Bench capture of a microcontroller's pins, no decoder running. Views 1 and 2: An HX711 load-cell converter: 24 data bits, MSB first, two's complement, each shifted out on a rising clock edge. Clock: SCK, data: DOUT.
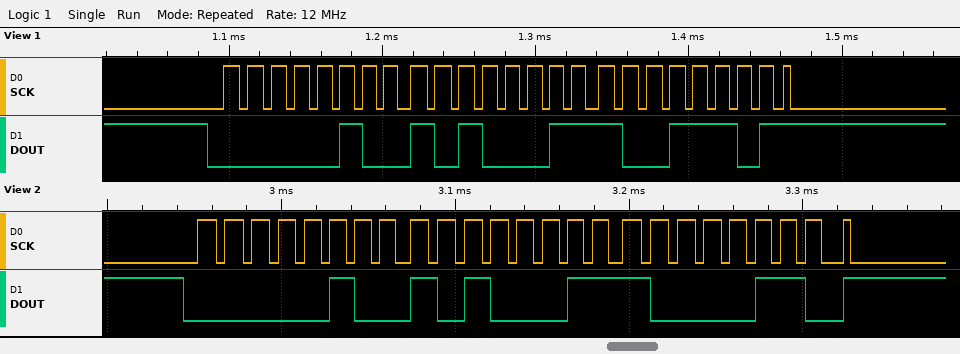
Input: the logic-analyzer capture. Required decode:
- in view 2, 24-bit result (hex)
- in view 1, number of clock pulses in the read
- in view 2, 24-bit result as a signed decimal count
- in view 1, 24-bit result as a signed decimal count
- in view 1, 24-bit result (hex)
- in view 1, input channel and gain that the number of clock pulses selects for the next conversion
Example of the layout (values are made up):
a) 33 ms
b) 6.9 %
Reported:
a) 0x04A386
b) 25
c) 304006
d) 304029
e) 0x04A39D
f) channel A, gain 128
